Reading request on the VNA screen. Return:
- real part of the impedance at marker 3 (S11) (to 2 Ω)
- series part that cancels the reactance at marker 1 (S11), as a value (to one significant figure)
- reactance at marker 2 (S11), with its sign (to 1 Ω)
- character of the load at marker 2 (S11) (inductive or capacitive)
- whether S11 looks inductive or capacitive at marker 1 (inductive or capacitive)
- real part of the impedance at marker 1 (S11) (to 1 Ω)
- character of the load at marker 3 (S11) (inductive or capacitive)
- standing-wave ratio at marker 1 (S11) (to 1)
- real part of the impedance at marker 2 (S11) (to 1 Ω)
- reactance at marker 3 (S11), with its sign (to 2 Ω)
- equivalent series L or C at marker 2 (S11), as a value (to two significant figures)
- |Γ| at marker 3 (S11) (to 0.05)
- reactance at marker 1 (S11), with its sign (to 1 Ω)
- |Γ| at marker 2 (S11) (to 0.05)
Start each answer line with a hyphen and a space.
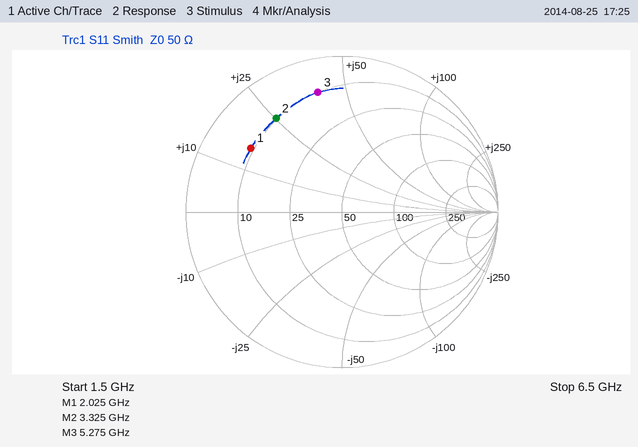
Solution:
- 10 Ω
- 5 pF
- +25 Ω
- inductive
- inductive
- 9 Ω
- inductive
- 6
- 10 Ω
- +40 Ω
- 1.2 nH
- 0.80
- +15 Ω
- 0.75
